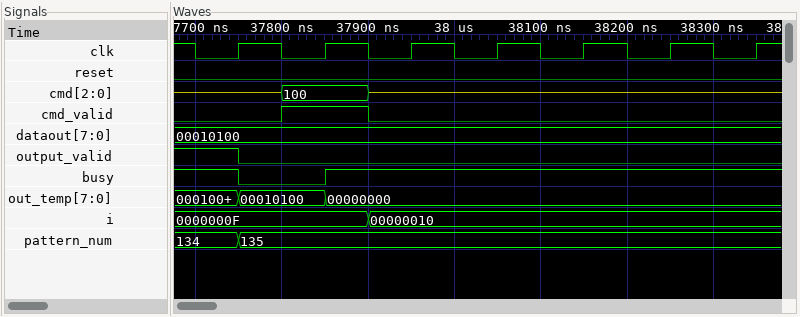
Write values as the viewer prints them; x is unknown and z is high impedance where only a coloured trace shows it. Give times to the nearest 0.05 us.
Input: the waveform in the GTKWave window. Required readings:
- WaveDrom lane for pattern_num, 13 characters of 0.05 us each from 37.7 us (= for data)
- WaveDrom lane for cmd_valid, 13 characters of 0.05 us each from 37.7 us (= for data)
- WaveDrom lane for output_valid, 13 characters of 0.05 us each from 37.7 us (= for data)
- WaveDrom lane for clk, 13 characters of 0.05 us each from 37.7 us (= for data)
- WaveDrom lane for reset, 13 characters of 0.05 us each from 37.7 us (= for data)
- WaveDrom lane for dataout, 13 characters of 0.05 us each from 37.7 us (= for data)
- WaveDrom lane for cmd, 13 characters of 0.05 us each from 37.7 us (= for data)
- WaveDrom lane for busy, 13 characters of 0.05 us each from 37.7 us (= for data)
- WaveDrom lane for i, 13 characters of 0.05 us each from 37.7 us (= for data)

{name: 'pattern_num', wave: '==...........', data: '134 135'}
{name: 'cmd_valid', wave: '0.1.0........'}
{name: 'output_valid', wave: '10...........'}
{name: 'clk', wave: '0101010101010'}
{name: 'reset', wave: '0............'}
{name: 'dataout', wave: '=............', data: '00010100'}
{name: 'cmd', wave: 'z.=.z........', data: '100'}
{name: 'busy', wave: '10.1.........'}
{name: 'i', wave: '=...=........', data: '0000000F 00000010'}
